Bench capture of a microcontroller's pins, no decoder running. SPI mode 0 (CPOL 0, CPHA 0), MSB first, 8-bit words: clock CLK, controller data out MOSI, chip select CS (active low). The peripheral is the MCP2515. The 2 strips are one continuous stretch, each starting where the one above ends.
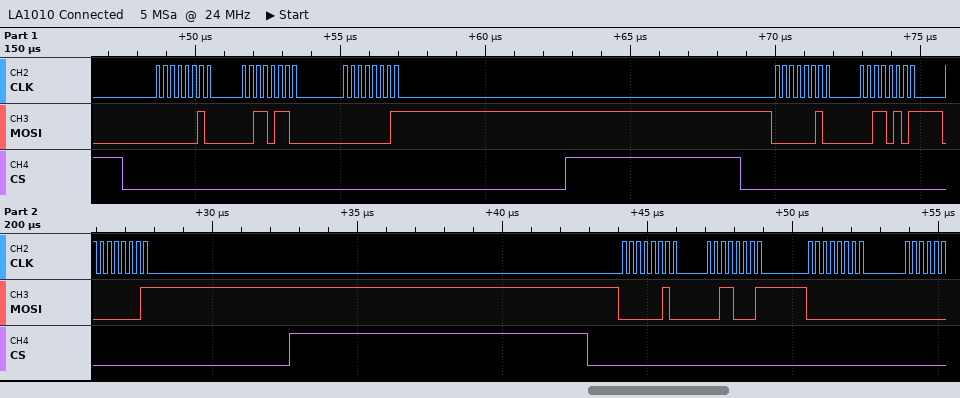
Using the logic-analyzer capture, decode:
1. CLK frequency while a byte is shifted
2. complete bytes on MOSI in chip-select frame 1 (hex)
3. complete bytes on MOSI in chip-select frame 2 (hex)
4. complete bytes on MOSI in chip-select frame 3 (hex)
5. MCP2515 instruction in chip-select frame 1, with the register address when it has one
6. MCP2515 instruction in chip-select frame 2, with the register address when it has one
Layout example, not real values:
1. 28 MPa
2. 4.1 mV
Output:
1. 4 MHz
2. 0x02 0x36 0x01
3. 0x02 0x35 0x01
4. 0x02 0x31 0x00
5. WRITE 0x36
6. WRITE 0x35
